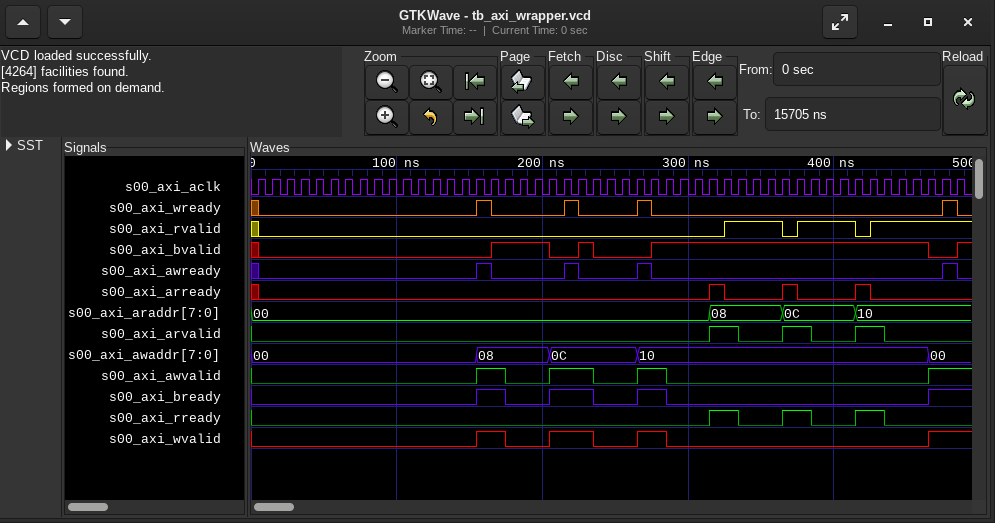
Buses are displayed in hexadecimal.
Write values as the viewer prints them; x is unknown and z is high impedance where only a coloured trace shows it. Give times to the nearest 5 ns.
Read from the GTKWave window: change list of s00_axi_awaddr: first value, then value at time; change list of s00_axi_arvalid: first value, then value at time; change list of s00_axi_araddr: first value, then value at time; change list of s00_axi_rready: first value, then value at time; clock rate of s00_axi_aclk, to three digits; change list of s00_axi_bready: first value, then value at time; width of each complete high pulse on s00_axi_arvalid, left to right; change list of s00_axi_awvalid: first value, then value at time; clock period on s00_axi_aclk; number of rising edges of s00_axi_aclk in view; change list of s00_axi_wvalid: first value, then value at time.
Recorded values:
00, 08 at 155 ns, 0C at 205 ns, 10 at 265 ns, 00 at 465 ns
0, 1 at 315 ns, 0 at 335 ns, 1 at 365 ns, 0 at 385 ns, 1 at 415 ns, 0 at 435 ns
00, 08 at 315 ns, 0C at 365 ns, 10 at 415 ns
0, 1 at 315 ns, 0 at 335 ns, 1 at 365 ns, 0 at 385 ns, 1 at 415 ns, 0 at 435 ns
100 MHz
0, 1 at 155 ns, 0 at 175 ns, 1 at 205 ns, 0 at 235 ns, 1 at 265 ns, 0 at 285 ns, 1 at 465 ns
20 ns, 20 ns, 20 ns
0, 1 at 155 ns, 0 at 175 ns, 1 at 205 ns, 0 at 235 ns, 1 at 265 ns, 0 at 285 ns, 1 at 465 ns
10 ns
49
0, 1 at 155 ns, 0 at 175 ns, 1 at 205 ns, 0 at 235 ns, 1 at 265 ns, 0 at 285 ns, 1 at 465 ns
